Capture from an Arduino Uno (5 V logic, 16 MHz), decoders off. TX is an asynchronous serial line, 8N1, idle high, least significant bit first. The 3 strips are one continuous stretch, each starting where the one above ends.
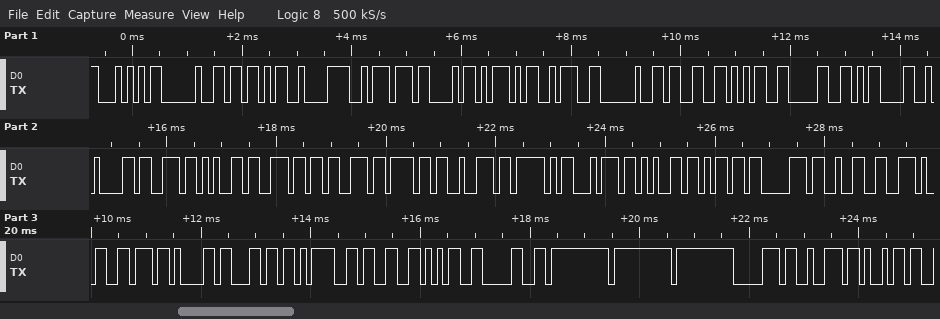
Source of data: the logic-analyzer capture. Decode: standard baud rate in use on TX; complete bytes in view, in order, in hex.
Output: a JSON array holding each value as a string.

["9600 baud", "54 20 5B C2 BA 43 5D 3A 20 33 35 30 0D 0A 73 65 6E 73 6F 72 5F 74 65 6D 70 32 2E 76 61 6C 3D 33 35 30 FF FF FF 70 72 69"]
